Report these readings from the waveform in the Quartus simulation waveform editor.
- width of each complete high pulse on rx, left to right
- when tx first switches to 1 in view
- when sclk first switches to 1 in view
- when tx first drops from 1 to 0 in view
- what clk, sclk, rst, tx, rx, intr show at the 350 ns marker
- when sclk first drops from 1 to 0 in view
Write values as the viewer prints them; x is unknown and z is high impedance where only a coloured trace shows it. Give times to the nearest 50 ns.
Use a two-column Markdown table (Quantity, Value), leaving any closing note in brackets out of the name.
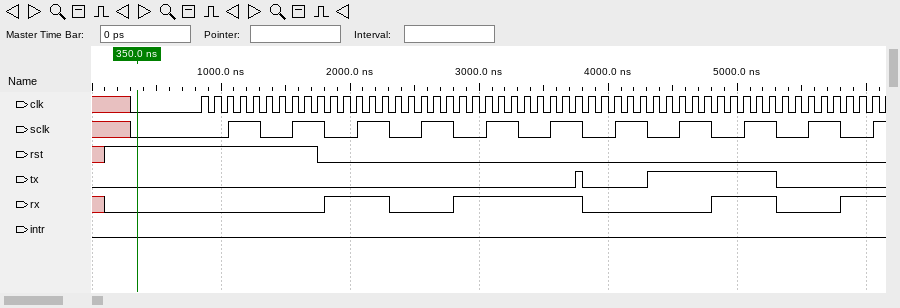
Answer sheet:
| Quantity | Value |
|---|---|
| width of each complete high pulse on rx, left to right | 500 ns, 1000 ns, 500 ns |
| when tx first switches to 1 in view | 3750 ns |
| when sclk first switches to 1 in view | 1050 ns |
| when tx first drops from 1 to 0 in view | 3800 ns |
| what clk, sclk, rst, tx, rx, intr show at the 350 ns marker | clk=0, sclk=0, rst=1, tx=0, rx=0, intr=0 |
| when sclk first drops from 1 to 0 in view | 1300 ns |
